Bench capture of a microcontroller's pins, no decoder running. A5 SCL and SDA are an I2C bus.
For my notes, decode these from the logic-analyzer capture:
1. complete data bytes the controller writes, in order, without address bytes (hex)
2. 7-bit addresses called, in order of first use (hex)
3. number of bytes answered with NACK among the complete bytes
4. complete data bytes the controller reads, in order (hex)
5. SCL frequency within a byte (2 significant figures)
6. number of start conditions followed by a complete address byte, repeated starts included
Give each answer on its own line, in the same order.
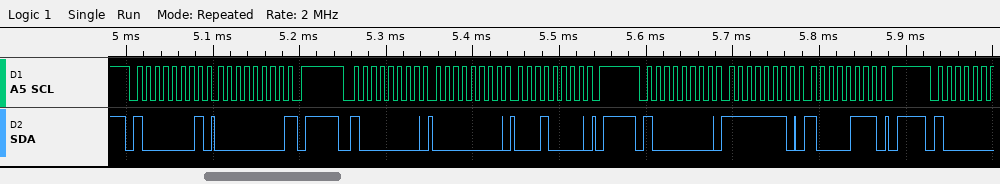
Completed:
00 10 FE 87
0x40
1
00
100 kHz
3
